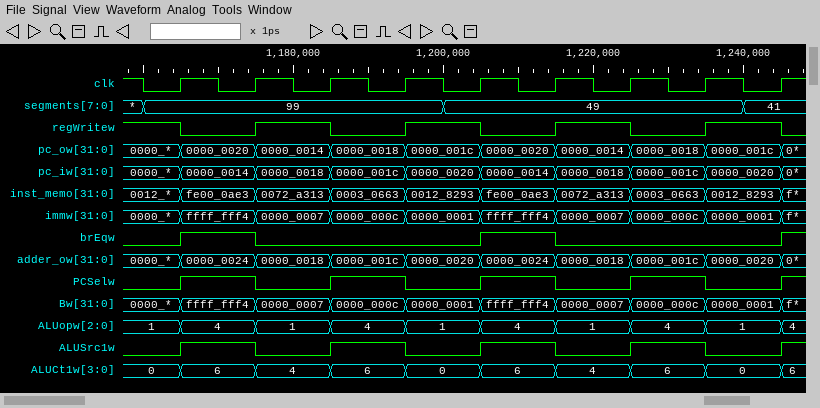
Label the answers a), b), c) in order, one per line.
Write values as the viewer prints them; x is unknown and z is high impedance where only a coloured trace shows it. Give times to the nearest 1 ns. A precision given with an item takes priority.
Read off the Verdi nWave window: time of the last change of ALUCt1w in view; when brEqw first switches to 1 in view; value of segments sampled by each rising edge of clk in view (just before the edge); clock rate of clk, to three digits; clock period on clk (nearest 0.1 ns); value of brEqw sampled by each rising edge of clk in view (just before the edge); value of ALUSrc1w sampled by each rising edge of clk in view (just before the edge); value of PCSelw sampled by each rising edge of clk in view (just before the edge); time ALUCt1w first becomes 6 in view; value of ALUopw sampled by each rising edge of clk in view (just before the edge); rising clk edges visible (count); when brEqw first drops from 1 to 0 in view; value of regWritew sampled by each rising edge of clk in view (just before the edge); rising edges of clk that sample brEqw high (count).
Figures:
a) 1245 ns
b) 1165 ns
c) 99, 99, 99, 99, 49, 49, 49, 49, 41
d) 100 MHz
e) 10 ns
f) 0 1 0 0 0 1 0 0 0
g) 0 1 0 1 0 1 0 1 0
h) 0 1 0 1 0 1 0 1 0
i) 1165 ns
j) 1, 4, 1, 4, 1, 4, 1, 4, 1
k) 9
l) 1175 ns
m) 1 0 1 0 1 0 1 0 1
n) 2
